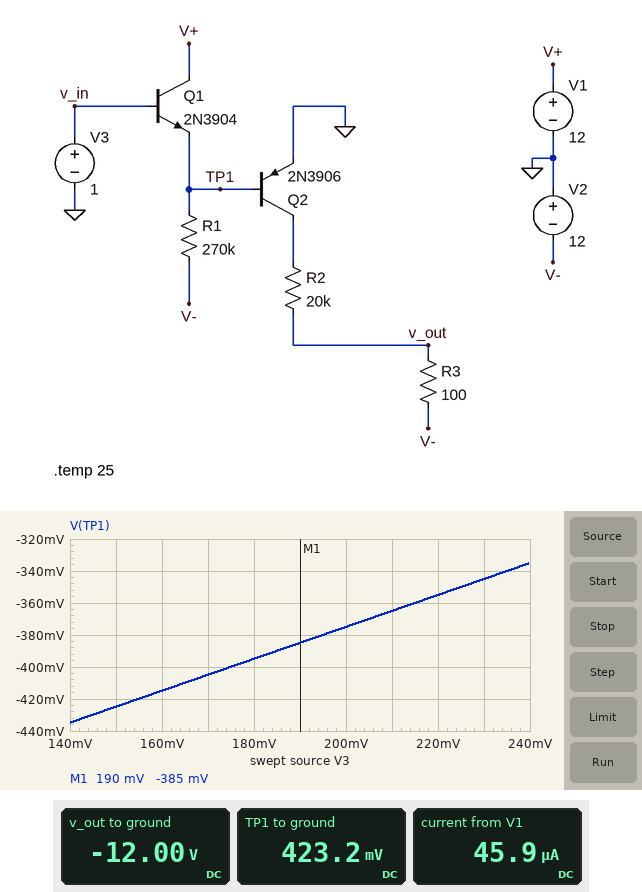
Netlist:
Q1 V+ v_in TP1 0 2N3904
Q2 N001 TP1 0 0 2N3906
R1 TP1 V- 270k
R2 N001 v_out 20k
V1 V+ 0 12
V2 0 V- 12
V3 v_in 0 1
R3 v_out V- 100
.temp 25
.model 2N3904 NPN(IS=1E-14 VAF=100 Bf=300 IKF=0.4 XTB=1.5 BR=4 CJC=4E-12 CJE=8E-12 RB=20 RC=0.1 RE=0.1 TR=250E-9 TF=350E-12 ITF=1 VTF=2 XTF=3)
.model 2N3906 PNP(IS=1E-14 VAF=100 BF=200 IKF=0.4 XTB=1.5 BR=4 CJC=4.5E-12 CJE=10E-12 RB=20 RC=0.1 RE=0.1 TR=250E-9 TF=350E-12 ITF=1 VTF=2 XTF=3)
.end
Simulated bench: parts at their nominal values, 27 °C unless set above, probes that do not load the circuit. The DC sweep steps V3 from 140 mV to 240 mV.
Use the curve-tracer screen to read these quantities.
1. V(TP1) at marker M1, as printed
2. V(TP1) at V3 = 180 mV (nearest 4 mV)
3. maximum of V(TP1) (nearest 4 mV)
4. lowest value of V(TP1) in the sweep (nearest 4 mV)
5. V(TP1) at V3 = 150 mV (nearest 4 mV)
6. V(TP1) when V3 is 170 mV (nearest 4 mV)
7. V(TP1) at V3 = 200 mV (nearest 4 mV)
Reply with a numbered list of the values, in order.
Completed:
1. -385 mV
2. -396 mV
3. -336 mV
4. -436 mV
5. -424 mV
6. -404 mV
7. -376 mV
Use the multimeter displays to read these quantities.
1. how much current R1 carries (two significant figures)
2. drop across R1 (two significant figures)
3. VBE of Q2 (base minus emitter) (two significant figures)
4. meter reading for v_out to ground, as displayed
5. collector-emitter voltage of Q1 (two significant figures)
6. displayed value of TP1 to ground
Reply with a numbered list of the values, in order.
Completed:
1. 46 µA
2. 12 V
3. 420 mV
4. -12.00 V
5. 12 V
6. 423.2 mV
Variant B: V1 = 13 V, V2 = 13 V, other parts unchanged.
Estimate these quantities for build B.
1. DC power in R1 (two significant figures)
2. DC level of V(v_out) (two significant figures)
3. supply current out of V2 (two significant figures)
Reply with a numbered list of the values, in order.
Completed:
1. 670 µW
2. -13 V
3. 50 µA
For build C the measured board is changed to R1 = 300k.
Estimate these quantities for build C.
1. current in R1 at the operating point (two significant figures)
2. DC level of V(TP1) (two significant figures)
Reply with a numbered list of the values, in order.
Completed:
1. 41 µA
2. 430 mV
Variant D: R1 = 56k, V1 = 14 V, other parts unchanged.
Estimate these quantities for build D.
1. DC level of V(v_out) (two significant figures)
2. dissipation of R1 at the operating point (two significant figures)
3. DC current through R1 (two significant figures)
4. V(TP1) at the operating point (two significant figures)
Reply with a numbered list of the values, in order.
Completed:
1. -12 V
2. 2.7 mW
3. 220 µA
4. 380 mV
